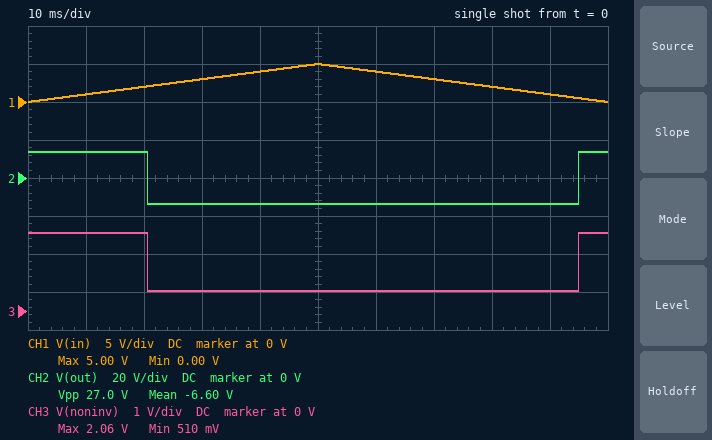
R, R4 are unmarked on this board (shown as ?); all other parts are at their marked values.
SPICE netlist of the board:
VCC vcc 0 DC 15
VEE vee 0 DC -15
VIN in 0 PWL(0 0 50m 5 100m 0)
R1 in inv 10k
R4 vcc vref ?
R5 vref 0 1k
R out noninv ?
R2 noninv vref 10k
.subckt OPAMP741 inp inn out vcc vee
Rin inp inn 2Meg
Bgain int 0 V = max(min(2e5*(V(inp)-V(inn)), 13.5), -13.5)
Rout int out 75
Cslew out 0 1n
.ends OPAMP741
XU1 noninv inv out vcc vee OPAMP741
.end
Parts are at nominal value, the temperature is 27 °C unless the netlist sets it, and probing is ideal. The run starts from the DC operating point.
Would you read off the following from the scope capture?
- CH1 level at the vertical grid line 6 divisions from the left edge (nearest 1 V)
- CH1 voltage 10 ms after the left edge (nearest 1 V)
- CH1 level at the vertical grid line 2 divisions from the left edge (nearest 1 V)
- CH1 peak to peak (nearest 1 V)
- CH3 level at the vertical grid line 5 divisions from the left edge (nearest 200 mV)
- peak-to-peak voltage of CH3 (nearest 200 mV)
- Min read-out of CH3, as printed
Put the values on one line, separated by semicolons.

4 V; 1 V; 2 V; 5 V; 600 mV; 1.6 V; 510 mV
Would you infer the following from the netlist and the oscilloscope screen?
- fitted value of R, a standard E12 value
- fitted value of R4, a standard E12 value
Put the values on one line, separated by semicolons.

180 kΩ; 10 kΩ
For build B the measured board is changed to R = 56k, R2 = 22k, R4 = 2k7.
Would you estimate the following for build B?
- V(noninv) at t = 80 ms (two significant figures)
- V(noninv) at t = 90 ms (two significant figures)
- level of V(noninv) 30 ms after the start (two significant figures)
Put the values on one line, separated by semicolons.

2.0 V; 1.0 V; 3.0 V
